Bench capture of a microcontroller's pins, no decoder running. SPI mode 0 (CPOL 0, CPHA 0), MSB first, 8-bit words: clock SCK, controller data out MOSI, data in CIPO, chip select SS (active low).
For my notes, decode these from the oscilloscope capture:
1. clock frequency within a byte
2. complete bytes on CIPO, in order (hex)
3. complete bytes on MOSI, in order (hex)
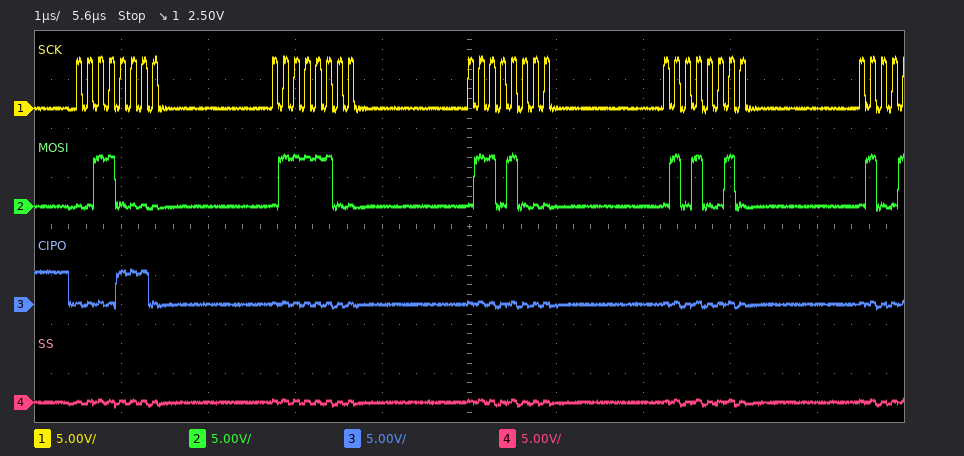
8 MHz
0x0E 0x00 0x00 0x00
0x30 0x7C 0x68 0x52
